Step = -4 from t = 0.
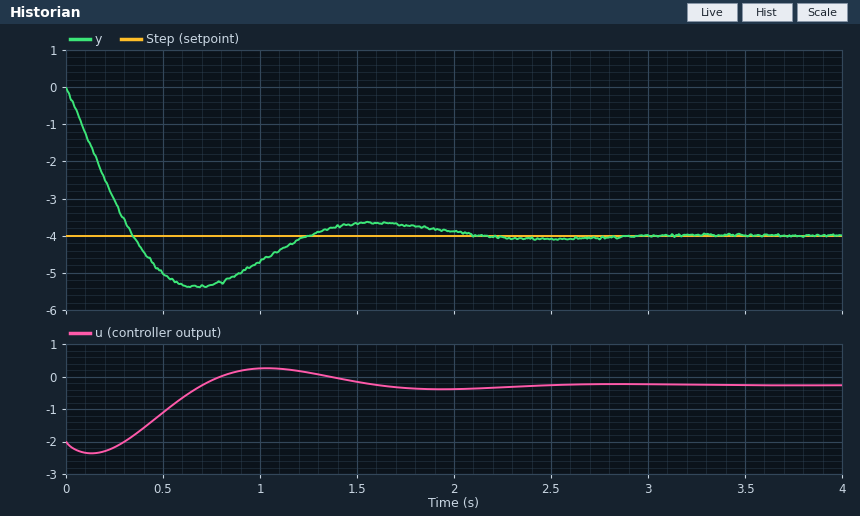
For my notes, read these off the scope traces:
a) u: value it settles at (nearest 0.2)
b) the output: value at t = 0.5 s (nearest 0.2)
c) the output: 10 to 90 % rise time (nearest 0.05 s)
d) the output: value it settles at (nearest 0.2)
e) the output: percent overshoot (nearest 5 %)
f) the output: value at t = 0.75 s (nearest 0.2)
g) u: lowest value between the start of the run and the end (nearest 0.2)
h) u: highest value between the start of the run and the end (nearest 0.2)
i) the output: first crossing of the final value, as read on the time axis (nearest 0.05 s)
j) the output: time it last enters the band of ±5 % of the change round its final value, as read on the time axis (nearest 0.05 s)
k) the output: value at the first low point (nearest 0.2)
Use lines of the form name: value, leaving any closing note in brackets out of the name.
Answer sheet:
u: value it settles at: -0.2
the output: value at t = 0.5 s: -5.0
the output: 10 to 90 % rise time: 0.25 s
the output: value it settles at: -4.0
the output: percent overshoot: 35 %
the output: value at t = 0.75 s: -5.4
u: lowest value between the start of the run and the end: -2.4
u: highest value between the start of the run and the end: 0.2
the output: first crossing of the final value, as read on the time axis: 0.35 s
the output: time it last enters the band of ±5 % of the change round its final value, as read on the time axis: 1.85 s
the output: value at the first low point: -5.4
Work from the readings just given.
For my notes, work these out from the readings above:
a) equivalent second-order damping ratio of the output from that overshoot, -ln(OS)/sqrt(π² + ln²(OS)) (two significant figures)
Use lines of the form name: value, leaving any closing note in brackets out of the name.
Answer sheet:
equivalent second-order damping ratio of the output from that overshoot, -ln(OS)/sqrt(π² + ln²(OS)): 0.32
